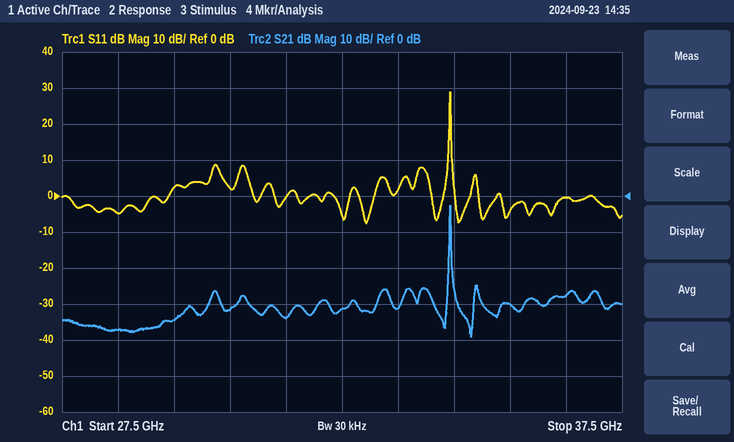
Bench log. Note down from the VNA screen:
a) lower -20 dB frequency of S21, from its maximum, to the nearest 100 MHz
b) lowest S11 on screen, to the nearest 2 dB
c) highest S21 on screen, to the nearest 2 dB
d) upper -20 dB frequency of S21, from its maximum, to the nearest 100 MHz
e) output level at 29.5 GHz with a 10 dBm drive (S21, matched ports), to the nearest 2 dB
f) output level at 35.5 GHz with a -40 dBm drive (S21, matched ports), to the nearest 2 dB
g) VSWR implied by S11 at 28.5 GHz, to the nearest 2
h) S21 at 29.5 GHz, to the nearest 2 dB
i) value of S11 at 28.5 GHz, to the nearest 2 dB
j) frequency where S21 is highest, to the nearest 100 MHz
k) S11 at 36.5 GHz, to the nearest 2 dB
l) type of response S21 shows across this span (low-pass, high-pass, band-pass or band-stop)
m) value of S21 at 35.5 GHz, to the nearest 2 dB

34.4 GHz
-8 dB
-2 dB
34.5 GHz
-24 dBm
-70 dBm
4
-34 dB
-4 dB
34.4 GHz
0 dB
band-pass
-30 dB
